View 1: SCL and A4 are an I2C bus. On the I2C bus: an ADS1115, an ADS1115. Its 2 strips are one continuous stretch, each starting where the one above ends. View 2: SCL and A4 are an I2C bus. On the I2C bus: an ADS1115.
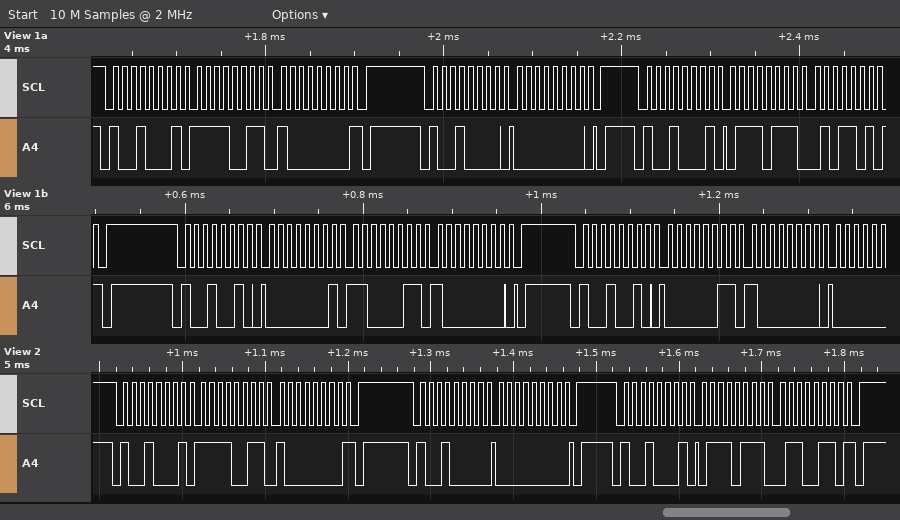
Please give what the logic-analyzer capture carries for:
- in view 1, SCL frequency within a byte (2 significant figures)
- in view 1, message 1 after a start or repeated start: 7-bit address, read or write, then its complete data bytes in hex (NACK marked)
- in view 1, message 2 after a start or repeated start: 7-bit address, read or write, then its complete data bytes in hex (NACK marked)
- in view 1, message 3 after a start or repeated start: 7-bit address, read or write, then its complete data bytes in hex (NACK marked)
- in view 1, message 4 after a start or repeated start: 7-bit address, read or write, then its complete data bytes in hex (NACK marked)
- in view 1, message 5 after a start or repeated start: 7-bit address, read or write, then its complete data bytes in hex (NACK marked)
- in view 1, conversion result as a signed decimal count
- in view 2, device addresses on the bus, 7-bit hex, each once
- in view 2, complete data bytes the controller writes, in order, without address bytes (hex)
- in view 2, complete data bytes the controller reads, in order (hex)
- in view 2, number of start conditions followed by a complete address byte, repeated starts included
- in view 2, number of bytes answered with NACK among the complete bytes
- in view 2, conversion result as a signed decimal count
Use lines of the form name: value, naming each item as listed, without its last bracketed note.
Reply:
in view 1, SCL frequency within a byte: 100 kHz
in view 1, message 1 after a start or repeated start: 7-bit address, read or write, then its complete data bytes in hex: 0x48 read: F3 80 NACK
in view 1, message 2 after a start or repeated start: 7-bit address, read or write, then its complete data bytes in hex: 0x48 write: 00
in view 1, message 3 after a start or repeated start: 7-bit address, read or write, then its complete data bytes in hex: 0x48 read: 77 5A NACK
in view 1, message 4 after a start or repeated start: 7-bit address, read or write, then its complete data bytes in hex: 0x49 write: 01 C3 80
in view 1, message 5 after a start or repeated start: 7-bit address, read or write, then its complete data bytes in hex: 0x49 write: 03 80
in view 1, conversion result as a signed decimal count: 30554
in view 2, device addresses on the bus, 7-bit hex, each once: 0x48
in view 2, complete data bytes the controller writes, in order, without address bytes: 00
in view 2, complete data bytes the controller reads, in order: F3 80 77 66
in view 2, number of start conditions followed by a complete address byte, repeated starts included: 3
in view 2, number of bytes answered with NACK among the complete bytes: 2
in view 2, conversion result as a signed decimal count: 30566
